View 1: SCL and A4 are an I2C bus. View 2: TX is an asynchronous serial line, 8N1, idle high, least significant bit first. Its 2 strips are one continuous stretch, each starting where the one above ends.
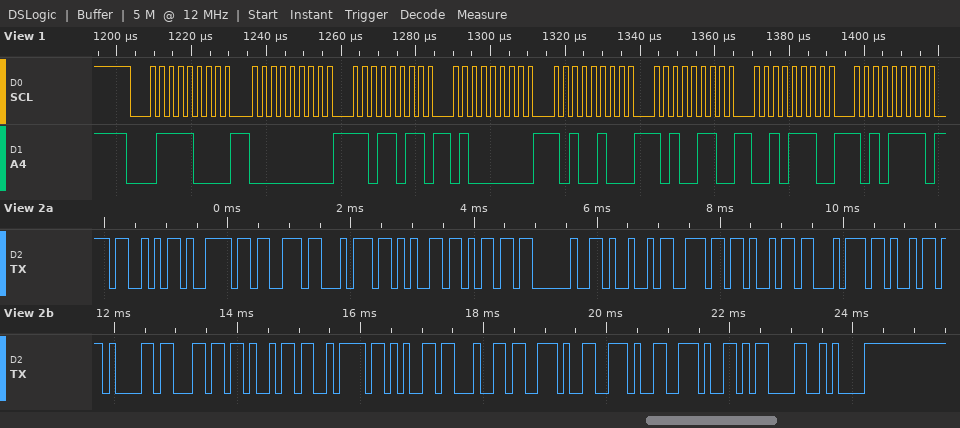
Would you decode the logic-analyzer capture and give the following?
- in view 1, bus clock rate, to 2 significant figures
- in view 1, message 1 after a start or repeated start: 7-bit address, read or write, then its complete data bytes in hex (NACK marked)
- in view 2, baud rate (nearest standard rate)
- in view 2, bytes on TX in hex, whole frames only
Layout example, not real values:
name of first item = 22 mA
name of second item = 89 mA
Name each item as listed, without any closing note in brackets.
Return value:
in view 1, bus clock rate, to 2 significant figures = 400 kHz
in view 1, message 1 after a start or repeated start: 7-bit address, read or write, then its complete data bytes in hex = 0x3C write: 00 DB 40 A4 A6 2E AF
in view 2, baud rate = 9600 baud
in view 2, bytes on TX in hex, whole frames only = 53 79 73 74 65 6D 20 49 6E 69 74 69 61 6C 69 7A 65 64 2E 2E 2E 0D 0A
